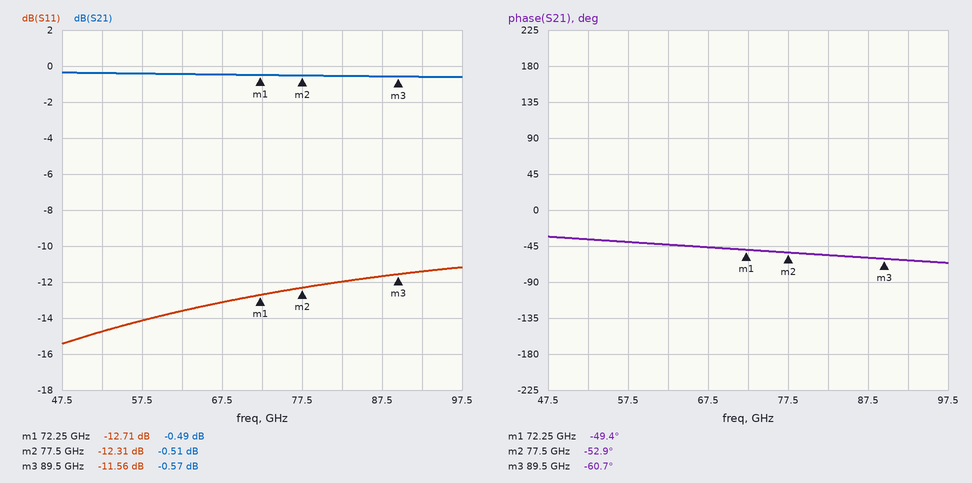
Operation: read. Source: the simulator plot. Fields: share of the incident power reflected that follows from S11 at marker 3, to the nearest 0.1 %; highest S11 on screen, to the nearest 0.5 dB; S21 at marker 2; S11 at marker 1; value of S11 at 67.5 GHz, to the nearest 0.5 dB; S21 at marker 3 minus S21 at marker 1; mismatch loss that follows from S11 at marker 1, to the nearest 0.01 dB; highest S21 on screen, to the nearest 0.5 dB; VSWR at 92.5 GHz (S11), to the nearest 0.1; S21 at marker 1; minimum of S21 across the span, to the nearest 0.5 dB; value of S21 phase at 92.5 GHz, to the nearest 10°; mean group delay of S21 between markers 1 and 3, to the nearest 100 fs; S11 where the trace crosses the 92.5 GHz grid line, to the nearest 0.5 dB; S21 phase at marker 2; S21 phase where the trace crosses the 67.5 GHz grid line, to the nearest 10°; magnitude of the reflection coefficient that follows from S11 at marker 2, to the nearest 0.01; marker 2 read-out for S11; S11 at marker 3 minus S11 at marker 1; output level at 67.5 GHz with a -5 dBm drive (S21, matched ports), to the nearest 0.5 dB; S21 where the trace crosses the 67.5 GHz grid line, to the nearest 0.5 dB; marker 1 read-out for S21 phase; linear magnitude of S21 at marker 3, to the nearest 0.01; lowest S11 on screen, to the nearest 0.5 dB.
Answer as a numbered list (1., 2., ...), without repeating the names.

1. 7.0 %
2. -11.0 dB
3. -0.51 dB
4. -12.71 dB
5. -13.0 dB
6. -0.08 dB
7. 0.24 dB
8. -0.5 dB
9. 1.7
10. -0.49 dB
11. -0.5 dB
12. -60°
13. 1.8 ps
14. -11.5 dB
15. -52.9°
16. -50°
17. 0.24
18. -12.31 dB
19. 1.15 dB
20. -5.5 dBm
21. -0.5 dB
22. -49.4°
23. 0.94
24. -15.5 dB
